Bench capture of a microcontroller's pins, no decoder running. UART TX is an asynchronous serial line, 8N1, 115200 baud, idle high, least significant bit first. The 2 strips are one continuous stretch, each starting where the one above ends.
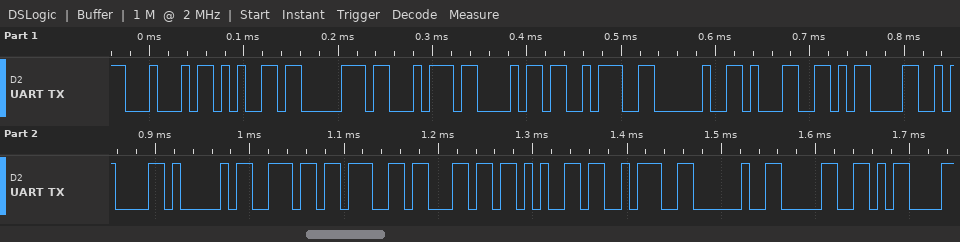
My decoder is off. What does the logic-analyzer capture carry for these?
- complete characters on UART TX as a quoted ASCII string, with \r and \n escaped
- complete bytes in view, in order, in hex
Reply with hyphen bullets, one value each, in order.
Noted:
- "Depth: 1\r\nAngle: 0\r"
- 44 65 70 74 68 3A 20 31 0D 0A 41 6E 67 6C 65 3A 20 30 0D
